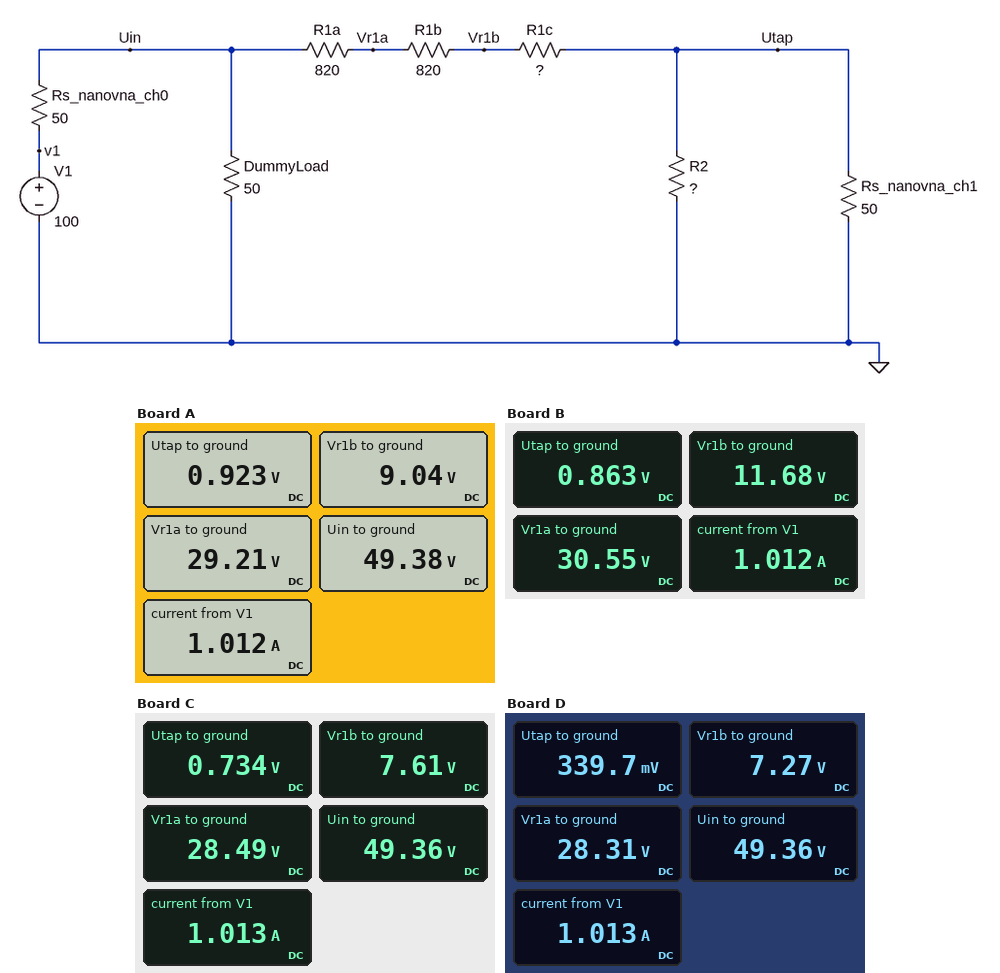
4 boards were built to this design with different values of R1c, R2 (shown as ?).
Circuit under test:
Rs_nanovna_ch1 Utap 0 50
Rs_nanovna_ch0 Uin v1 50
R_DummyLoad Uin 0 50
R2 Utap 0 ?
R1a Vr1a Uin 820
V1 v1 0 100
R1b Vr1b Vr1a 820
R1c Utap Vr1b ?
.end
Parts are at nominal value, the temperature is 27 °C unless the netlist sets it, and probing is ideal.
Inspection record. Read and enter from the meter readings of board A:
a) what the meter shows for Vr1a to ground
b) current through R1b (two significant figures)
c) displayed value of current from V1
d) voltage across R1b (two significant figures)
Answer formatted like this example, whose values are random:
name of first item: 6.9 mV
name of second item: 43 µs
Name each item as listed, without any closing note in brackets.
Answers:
what the meter shows for Vr1a to ground: 29.21 V
current through R1b: 25 mA
displayed value of current from V1: 1.012 A
voltage across R1b: 20 V
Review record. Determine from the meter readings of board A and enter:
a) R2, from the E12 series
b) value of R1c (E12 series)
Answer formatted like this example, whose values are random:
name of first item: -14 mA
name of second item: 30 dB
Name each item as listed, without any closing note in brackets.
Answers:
R2, from the E12 series: 150 Ω
value of R1c: 330 Ω
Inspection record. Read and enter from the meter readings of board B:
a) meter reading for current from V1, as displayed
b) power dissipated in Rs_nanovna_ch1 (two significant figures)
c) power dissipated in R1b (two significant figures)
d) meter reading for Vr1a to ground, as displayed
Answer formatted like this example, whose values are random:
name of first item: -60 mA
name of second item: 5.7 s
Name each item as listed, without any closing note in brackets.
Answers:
meter reading for current from V1, as displayed: 1.012 A
power dissipated in Rs_nanovna_ch1: 15 mW
power dissipated in R1b: 430 mW
meter reading for Vr1a to ground, as displayed: 30.55 V
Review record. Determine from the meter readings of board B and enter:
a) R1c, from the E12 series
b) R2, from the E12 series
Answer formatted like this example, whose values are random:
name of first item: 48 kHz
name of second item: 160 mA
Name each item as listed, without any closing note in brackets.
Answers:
R1c, from the E12 series: 470 Ω
R2, from the E12 series: 150 Ω
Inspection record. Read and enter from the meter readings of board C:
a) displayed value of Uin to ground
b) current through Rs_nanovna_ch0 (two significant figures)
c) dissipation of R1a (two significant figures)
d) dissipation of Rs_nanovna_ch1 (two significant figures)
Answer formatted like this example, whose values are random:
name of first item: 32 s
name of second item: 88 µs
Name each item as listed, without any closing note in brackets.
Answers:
displayed value of Uin to ground: 49.36 V
current through Rs_nanovna_ch0: 1.0 A
dissipation of R1a: 530 mW
dissipation of Rs_nanovna_ch1: 11 mW
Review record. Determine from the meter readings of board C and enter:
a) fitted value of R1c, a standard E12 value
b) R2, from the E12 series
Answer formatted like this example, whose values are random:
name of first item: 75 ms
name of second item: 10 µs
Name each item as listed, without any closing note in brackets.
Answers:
fitted value of R1c, a standard E12 value: 270 Ω
R2, from the E12 series: 68 Ω
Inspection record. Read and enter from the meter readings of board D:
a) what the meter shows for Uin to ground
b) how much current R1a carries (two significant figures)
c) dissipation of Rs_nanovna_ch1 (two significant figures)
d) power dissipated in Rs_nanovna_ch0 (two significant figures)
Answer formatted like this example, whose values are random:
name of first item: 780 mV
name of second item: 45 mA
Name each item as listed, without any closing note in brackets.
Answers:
what the meter shows for Uin to ground: 49.36 V
how much current R1a carries: 26 mA
dissipation of Rs_nanovna_ch1: 2.3 mW
power dissipated in Rs_nanovna_ch0: 51 W
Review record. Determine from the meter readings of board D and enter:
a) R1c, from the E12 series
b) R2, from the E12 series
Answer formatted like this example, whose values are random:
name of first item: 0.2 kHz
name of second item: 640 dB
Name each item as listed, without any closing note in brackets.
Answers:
R1c, from the E12 series: 270 Ω
R2, from the E12 series: 18 Ω
